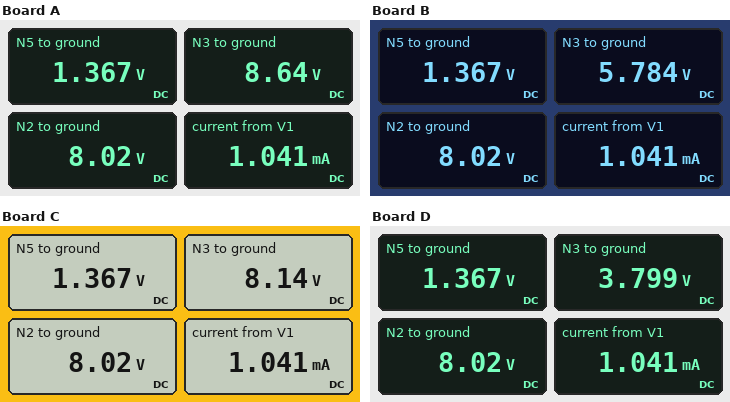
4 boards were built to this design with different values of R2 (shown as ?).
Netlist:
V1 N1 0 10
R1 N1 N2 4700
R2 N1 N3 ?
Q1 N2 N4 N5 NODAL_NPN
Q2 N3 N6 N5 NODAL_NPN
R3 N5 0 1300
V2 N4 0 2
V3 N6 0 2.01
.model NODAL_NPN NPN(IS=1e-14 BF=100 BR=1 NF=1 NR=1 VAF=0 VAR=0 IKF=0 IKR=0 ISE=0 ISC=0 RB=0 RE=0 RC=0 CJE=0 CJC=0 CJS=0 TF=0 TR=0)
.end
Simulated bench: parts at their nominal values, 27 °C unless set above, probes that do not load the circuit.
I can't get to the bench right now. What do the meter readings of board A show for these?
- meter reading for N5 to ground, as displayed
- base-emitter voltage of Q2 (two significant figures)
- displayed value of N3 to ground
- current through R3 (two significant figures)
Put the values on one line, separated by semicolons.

1.367 V; 640 mV; 8.64 V; 1.1 mA
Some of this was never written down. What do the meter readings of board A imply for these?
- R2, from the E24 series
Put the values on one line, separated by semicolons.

2.2 kΩ
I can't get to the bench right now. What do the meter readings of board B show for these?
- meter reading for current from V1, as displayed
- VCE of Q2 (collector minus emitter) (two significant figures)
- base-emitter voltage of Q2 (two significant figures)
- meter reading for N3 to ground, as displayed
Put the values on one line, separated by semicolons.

1.041 mA; 4.4 V; 640 mV; 5.784 V
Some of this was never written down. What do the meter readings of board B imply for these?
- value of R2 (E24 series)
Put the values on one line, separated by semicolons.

6.8 kΩ
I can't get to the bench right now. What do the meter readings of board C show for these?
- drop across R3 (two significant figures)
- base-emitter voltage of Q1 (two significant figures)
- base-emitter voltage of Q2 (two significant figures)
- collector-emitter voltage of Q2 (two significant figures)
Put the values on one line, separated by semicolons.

1.4 V; 630 mV; 640 mV; 6.8 V
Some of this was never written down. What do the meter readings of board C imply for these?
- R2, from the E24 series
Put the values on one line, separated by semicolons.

3 kΩ
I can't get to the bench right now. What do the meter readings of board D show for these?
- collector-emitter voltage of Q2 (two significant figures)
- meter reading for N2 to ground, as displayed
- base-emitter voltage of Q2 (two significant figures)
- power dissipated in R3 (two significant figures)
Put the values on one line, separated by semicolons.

2.4 V; 8.02 V; 640 mV; 1.4 mW
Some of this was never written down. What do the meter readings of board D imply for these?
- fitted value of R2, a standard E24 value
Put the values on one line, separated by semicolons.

10 kΩ
